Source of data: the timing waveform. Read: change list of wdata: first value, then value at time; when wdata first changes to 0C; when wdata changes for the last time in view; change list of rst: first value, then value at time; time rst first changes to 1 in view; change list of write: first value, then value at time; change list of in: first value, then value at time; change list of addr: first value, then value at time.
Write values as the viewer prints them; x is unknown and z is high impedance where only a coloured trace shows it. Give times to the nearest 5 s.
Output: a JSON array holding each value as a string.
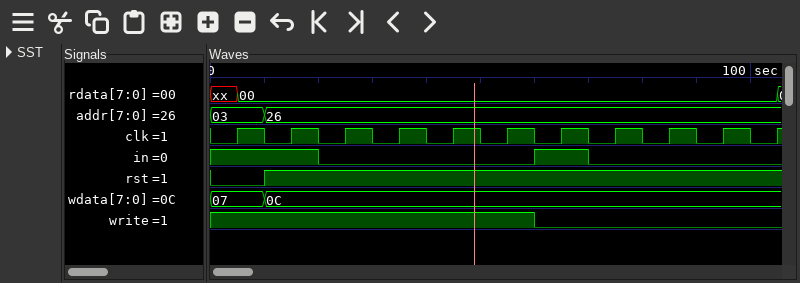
["07, 0C at 10 s", "10 s", "10 s", "0, 1 at 10 s", "10 s", "1, 0 at 60 s", "1, 0 at 20 s, 1 at 60 s, 0 at 70 s", "03, 26 at 10 s"]
